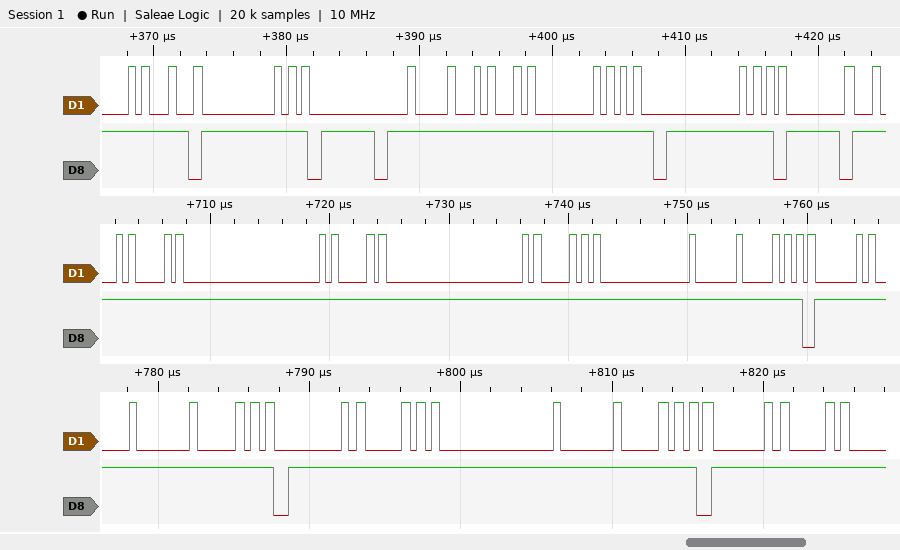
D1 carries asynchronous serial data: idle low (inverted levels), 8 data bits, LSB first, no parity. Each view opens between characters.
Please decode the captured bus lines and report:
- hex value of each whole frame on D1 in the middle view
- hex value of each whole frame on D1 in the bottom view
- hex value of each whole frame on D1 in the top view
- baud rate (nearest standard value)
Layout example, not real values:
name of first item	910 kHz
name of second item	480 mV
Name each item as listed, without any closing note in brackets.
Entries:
hex value of each whole frame on D1 in the middle view	7D, FF, 7D, FF, 7D, FD, 7F, D5
hex value of each whole frame on D1 in the bottom view	7F, F5, 7D, FD, 7F, D5, 7D
hex value of each whole frame on D1 in the top view	DD, FF, F5, DF, 5D, D5, D5
baud rate	2000000 baud
